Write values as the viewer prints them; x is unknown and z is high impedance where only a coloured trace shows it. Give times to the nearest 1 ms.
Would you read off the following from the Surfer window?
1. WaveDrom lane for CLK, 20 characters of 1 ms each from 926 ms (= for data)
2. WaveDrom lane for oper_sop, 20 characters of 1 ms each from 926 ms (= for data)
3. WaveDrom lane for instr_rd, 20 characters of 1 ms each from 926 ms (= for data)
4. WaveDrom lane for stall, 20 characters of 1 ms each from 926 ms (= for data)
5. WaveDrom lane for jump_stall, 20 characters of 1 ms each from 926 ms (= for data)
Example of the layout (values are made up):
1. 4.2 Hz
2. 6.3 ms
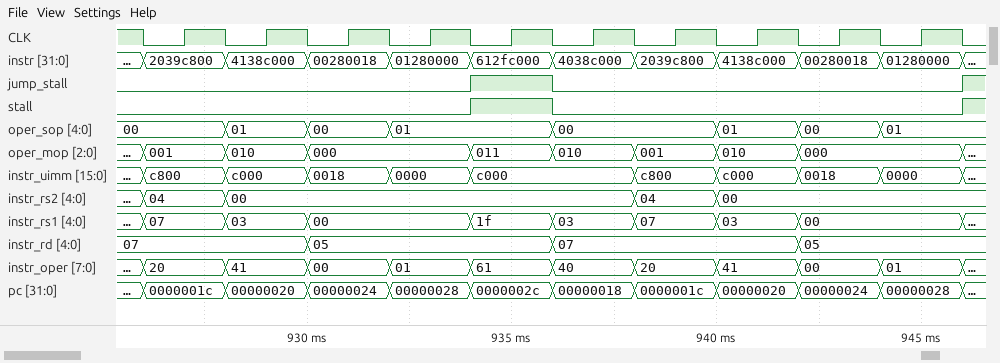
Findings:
1. {name: 'CLK', wave: '01010101010101010101'}
2. {name: 'oper_sop', wave: '=.=.=.=...=...=.=.=.', data: '00 01 00 01 00 01 00 01'}
3. {name: 'instr_rd', wave: '=...=.....=.....=...', data: '07 05 07 05'}
4. {name: 'stall', wave: '0.......1.0.........'}
5. {name: 'jump_stall', wave: '0.......1.0.........'}
